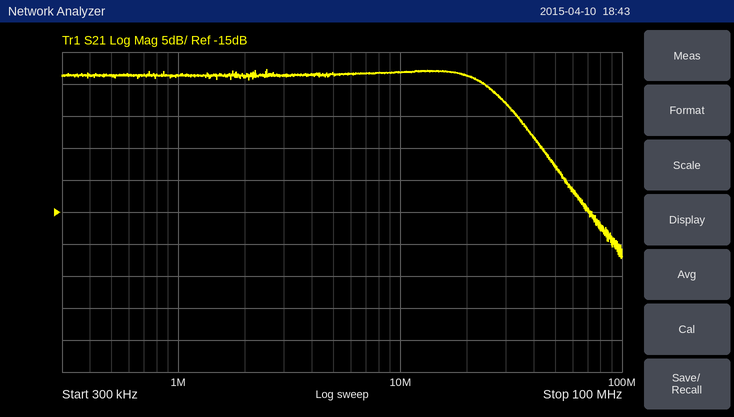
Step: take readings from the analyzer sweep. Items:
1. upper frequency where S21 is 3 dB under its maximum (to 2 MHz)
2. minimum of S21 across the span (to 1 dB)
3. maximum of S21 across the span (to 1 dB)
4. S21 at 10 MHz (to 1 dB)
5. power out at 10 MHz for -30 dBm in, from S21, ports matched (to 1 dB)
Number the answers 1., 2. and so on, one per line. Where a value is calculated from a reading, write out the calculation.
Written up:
1. 26 MHz
2. -22 dB
3. 7 dB
4. 7 dB
5. -30 dBm + (7 dB) = -23 dBm
